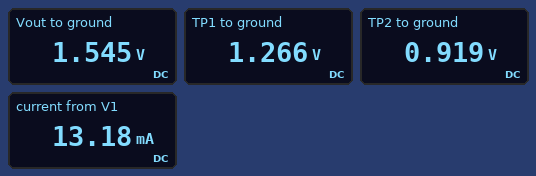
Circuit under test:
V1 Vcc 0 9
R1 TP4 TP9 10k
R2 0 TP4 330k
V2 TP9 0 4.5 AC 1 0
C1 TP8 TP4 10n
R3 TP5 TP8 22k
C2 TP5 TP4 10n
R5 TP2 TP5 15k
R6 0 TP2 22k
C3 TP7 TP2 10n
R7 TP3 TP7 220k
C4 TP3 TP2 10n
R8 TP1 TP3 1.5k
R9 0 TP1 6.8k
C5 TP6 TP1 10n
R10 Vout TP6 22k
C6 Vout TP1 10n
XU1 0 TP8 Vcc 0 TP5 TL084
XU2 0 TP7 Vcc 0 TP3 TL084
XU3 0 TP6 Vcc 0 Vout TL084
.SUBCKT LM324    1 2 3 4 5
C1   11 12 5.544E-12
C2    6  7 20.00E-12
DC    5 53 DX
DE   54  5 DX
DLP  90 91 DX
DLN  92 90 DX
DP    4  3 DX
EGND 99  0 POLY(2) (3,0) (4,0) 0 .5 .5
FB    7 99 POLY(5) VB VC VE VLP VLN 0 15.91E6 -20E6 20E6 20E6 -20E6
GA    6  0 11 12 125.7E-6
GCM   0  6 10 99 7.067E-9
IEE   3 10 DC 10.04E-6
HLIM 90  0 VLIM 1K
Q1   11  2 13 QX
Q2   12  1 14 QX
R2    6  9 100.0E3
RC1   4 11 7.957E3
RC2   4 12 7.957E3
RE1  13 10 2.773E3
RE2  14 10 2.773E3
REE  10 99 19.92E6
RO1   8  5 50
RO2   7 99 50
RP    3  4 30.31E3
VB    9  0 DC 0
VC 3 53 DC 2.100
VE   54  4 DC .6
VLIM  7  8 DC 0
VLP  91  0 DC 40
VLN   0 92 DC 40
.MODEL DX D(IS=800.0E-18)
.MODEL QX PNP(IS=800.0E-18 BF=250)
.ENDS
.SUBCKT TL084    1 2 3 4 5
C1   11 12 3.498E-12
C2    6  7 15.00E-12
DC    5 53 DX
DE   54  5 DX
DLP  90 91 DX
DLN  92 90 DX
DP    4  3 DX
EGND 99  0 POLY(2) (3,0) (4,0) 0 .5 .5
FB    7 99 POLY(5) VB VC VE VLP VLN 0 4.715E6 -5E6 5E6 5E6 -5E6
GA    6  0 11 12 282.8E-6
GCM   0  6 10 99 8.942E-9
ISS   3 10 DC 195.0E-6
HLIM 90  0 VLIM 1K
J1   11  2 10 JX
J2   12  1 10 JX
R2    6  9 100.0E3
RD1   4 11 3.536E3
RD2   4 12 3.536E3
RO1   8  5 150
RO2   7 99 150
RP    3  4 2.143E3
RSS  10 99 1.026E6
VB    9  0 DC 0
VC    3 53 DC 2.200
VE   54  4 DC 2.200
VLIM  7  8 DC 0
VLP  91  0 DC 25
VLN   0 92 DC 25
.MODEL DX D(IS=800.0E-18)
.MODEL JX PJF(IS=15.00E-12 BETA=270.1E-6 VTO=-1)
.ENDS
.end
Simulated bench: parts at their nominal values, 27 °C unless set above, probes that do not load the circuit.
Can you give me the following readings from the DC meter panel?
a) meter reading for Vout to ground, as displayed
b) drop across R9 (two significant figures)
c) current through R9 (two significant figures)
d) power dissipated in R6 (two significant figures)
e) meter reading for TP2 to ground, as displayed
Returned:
1.545 V
1.3 V
190 µA
38 µW
0.919 V
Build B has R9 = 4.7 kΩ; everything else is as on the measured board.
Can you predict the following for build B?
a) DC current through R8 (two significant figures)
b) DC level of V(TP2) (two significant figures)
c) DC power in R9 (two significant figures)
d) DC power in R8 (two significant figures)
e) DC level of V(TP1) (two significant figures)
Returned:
250 µA
920 mV
290 µW
93 µW
1.2 V
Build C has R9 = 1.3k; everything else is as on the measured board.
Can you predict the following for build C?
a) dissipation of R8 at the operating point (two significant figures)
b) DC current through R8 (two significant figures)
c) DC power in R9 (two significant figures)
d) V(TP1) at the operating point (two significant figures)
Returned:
460 µW
550 µA
400 µW
720 mV
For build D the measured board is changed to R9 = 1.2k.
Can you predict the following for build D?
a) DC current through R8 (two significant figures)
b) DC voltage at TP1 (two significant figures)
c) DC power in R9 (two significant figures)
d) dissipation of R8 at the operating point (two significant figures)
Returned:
570 µA
690 mV
390 µW
490 µW
